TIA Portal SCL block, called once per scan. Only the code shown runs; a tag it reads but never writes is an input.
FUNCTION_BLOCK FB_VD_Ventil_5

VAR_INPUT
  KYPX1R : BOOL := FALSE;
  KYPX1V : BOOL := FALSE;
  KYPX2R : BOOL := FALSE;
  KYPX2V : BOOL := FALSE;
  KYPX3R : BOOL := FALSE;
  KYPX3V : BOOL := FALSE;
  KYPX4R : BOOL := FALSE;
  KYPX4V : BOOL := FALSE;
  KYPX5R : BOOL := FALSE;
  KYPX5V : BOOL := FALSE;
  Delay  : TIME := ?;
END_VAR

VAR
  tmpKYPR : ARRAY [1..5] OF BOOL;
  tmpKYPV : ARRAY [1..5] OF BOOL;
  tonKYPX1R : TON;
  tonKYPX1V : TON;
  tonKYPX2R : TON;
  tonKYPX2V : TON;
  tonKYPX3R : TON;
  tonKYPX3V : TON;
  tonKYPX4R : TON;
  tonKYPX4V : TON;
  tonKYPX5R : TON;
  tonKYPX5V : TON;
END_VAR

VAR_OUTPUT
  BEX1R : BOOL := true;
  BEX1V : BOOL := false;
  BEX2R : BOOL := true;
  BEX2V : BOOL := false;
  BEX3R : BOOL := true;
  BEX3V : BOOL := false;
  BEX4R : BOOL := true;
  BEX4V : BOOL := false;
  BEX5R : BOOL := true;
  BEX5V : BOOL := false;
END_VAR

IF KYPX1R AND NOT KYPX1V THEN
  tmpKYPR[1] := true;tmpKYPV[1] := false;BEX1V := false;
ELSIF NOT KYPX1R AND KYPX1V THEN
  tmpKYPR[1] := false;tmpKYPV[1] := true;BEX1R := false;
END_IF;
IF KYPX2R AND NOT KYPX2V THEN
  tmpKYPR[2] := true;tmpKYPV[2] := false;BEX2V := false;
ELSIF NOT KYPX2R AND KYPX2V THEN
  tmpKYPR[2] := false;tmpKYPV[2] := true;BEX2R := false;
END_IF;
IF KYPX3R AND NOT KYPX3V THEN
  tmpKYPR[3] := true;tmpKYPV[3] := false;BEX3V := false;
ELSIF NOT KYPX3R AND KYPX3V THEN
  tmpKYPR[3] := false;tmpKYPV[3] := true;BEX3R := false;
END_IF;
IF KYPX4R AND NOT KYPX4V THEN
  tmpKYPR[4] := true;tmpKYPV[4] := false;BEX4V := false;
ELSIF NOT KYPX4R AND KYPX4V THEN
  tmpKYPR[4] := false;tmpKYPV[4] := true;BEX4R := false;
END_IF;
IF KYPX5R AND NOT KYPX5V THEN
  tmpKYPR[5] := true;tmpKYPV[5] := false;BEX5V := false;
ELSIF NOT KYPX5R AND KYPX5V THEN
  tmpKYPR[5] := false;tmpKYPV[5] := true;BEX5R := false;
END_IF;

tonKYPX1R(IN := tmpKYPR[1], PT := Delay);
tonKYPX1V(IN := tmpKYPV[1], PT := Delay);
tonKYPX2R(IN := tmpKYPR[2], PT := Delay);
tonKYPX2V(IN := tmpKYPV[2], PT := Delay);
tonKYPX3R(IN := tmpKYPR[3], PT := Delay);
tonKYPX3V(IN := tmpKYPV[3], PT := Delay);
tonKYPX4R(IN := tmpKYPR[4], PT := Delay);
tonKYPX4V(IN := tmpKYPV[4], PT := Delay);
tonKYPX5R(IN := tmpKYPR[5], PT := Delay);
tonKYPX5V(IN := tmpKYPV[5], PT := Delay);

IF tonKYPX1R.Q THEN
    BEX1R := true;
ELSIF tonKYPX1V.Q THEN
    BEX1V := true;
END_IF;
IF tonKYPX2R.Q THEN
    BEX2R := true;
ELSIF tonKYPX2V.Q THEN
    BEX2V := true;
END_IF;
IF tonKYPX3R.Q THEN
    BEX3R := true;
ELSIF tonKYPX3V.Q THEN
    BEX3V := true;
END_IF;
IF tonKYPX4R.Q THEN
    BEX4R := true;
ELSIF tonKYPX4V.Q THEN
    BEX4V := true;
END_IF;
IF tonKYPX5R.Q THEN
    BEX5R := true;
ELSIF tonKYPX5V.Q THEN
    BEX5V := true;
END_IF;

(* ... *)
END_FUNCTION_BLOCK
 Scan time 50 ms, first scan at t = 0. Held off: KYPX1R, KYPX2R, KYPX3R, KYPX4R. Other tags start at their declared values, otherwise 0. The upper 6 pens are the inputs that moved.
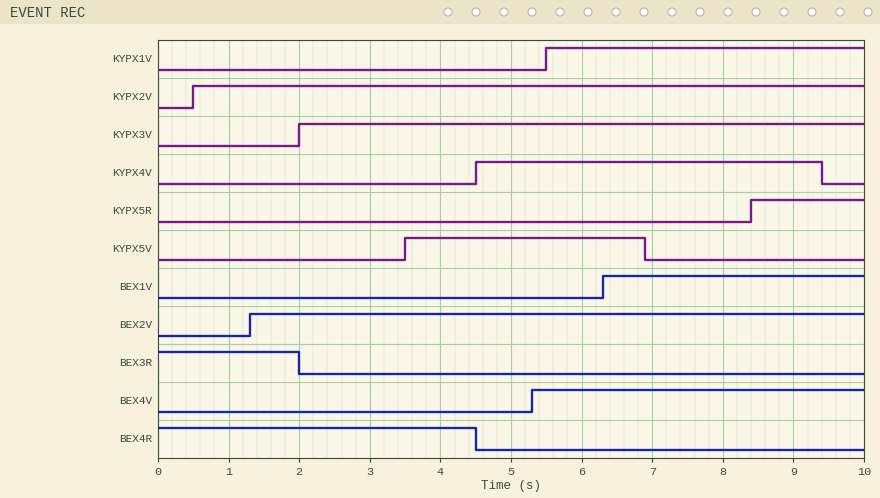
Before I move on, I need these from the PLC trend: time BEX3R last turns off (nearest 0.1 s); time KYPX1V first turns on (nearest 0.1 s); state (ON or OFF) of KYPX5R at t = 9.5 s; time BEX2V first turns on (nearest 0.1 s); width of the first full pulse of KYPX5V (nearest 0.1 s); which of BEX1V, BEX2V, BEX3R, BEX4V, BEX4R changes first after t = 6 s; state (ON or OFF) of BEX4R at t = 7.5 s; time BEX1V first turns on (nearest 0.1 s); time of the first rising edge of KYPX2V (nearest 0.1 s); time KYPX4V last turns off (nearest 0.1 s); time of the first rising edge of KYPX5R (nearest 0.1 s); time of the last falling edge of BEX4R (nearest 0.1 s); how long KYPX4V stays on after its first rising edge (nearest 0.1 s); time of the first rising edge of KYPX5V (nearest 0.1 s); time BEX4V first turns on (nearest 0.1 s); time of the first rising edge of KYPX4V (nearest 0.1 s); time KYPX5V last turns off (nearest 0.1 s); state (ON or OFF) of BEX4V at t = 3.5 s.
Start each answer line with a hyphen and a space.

- 2.0 s
- 5.5 s
- ON
- 1.3 s
- 3.4 s
- BEX1V
- OFF
- 6.3 s
- 0.5 s
- 9.4 s
- 8.4 s
- 4.5 s
- 4.9 s
- 3.5 s
- 5.3 s
- 4.5 s
- 6.9 s
- OFF
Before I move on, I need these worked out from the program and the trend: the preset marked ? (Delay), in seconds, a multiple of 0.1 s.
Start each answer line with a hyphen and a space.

- 0.8 s
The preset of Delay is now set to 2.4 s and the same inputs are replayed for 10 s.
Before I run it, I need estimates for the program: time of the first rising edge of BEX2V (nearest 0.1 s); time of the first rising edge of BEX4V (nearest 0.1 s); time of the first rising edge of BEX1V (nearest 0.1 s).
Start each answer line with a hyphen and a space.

- 2.9 s
- 6.9 s
- 7.9 s
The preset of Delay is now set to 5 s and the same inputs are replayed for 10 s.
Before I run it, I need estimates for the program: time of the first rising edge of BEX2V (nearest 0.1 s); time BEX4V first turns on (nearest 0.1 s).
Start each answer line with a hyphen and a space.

- 5.5 s
- 9.5 s
